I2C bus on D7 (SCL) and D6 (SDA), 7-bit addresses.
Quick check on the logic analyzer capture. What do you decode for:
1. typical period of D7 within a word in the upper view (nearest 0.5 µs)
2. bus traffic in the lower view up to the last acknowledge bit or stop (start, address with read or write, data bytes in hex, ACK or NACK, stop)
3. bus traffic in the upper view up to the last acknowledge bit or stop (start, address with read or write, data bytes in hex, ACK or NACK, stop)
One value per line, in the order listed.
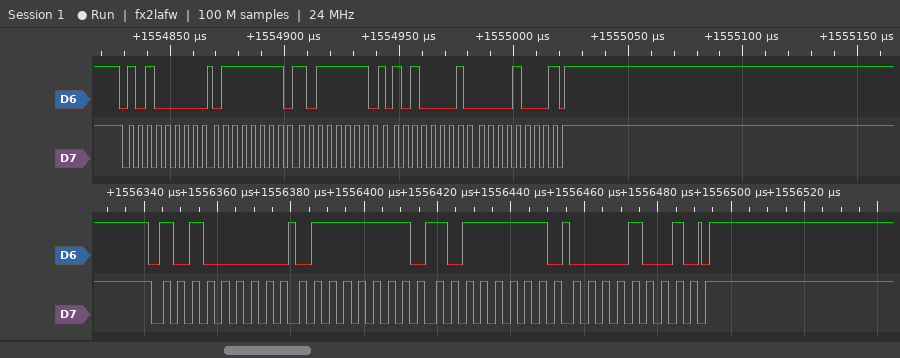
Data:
4 µs
start, address 50 write ACK, 7F ACK, BF ACK, 09 ACK, stop
start, address 50 write ACK, 7F ACK, BF ACK, repeated start, address 50 read ACK, 08 NACK, stop
